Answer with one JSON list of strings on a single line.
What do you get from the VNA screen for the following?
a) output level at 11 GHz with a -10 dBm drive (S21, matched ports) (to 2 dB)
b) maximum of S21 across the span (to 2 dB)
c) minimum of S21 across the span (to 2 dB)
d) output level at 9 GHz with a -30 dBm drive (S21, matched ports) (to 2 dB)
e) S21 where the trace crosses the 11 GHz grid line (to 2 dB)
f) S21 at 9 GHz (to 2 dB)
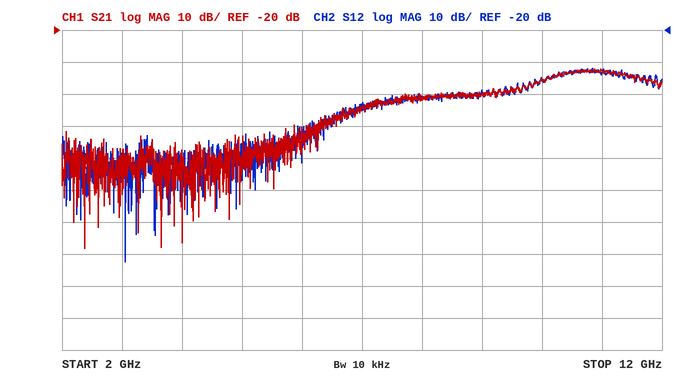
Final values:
["-42 dBm", "-32 dB", "-88 dB", "-70 dBm", "-32 dB", "-40 dB"]
